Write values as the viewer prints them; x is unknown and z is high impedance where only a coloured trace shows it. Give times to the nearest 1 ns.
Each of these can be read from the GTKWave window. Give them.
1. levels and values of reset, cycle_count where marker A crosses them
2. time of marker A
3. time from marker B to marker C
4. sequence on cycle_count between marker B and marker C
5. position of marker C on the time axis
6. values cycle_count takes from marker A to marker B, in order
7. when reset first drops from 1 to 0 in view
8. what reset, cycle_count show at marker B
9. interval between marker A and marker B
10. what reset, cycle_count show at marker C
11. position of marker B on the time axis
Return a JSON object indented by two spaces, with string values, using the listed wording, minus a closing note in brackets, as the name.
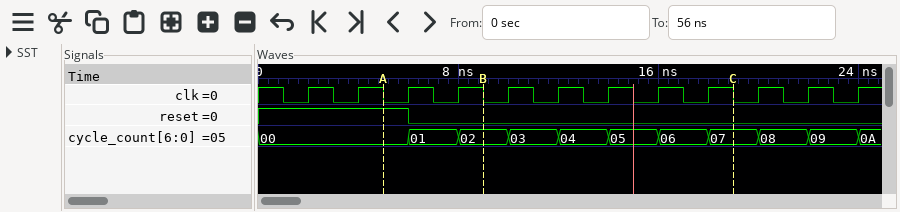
{
  "levels and values of reset, cycle_count where marker A crosses them": "reset=1, cycle_count=00",
  "time of marker A": "5 ns",
  "time from marker B to marker C": "10 ns",
  "sequence on cycle_count between marker B and marker C": "02, 03, 04, 05, 06, 07",
  "position of marker C on the time axis": "19 ns",
  "values cycle_count takes from marker A to marker B, in order": "00, 01, 02",
  "when reset first drops from 1 to 0 in view": "6 ns",
  "what reset, cycle_count show at marker B": "reset=0, cycle_count=02",
  "interval between marker A and marker B": "4 ns",
  "what reset, cycle_count show at marker C": "reset=0, cycle_count=07",
  "position of marker B on the time axis": "9 ns"
}
